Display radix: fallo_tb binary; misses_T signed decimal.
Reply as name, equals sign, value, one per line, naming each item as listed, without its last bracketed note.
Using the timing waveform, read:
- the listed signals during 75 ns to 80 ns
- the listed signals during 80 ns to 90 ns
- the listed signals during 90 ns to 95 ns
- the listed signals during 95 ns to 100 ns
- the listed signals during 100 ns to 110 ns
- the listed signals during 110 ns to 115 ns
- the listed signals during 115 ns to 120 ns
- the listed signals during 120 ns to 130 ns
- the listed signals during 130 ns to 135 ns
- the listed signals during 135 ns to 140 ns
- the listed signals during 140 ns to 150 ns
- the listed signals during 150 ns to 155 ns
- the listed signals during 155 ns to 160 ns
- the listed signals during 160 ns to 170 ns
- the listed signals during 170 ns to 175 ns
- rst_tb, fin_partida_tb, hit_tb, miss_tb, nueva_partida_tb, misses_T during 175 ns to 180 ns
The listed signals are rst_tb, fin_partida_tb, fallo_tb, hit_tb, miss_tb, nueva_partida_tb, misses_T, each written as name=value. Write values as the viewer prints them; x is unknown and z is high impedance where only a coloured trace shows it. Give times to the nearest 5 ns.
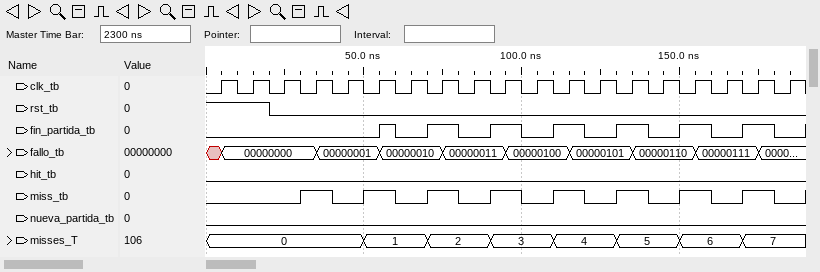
the listed signals during 75 ns to 80 ns = rst_tb=0, fin_partida_tb=1, fallo_tb=00000011, hit_tb=0, miss_tb=1, nueva_partida_tb=0, misses_T=2
the listed signals during 80 ns to 90 ns = rst_tb=0, fin_partida_tb=0, fallo_tb=00000011, hit_tb=0, miss_tb=0, nueva_partida_tb=0, misses_T=2
the listed signals during 90 ns to 95 ns = rst_tb=0, fin_partida_tb=1, fallo_tb=00000011, hit_tb=0, miss_tb=1, nueva_partida_tb=0, misses_T=3
the listed signals during 95 ns to 100 ns = rst_tb=0, fin_partida_tb=1, fallo_tb=00000100, hit_tb=0, miss_tb=1, nueva_partida_tb=0, misses_T=3
the listed signals during 100 ns to 110 ns = rst_tb=0, fin_partida_tb=0, fallo_tb=00000100, hit_tb=0, miss_tb=0, nueva_partida_tb=0, misses_T=3
the listed signals during 110 ns to 115 ns = rst_tb=0, fin_partida_tb=1, fallo_tb=00000100, hit_tb=0, miss_tb=1, nueva_partida_tb=0, misses_T=4
the listed signals during 115 ns to 120 ns = rst_tb=0, fin_partida_tb=1, fallo_tb=00000101, hit_tb=0, miss_tb=1, nueva_partida_tb=0, misses_T=4
the listed signals during 120 ns to 130 ns = rst_tb=0, fin_partida_tb=0, fallo_tb=00000101, hit_tb=0, miss_tb=0, nueva_partida_tb=0, misses_T=4
the listed signals during 130 ns to 135 ns = rst_tb=0, fin_partida_tb=1, fallo_tb=00000101, hit_tb=0, miss_tb=1, nueva_partida_tb=0, misses_T=5
the listed signals during 135 ns to 140 ns = rst_tb=0, fin_partida_tb=1, fallo_tb=00000110, hit_tb=0, miss_tb=1, nueva_partida_tb=0, misses_T=5
the listed signals during 140 ns to 150 ns = rst_tb=0, fin_partida_tb=0, fallo_tb=00000110, hit_tb=0, miss_tb=0, nueva_partida_tb=0, misses_T=5
the listed signals during 150 ns to 155 ns = rst_tb=0, fin_partida_tb=1, fallo_tb=00000110, hit_tb=0, miss_tb=1, nueva_partida_tb=0, misses_T=6
the listed signals during 155 ns to 160 ns = rst_tb=0, fin_partida_tb=1, fallo_tb=00000111, hit_tb=0, miss_tb=1, nueva_partida_tb=0, misses_T=6
the listed signals during 160 ns to 170 ns = rst_tb=0, fin_partida_tb=0, fallo_tb=00000111, hit_tb=0, miss_tb=0, nueva_partida_tb=0, misses_T=6
the listed signals during 170 ns to 175 ns = rst_tb=0, fin_partida_tb=1, fallo_tb=00000111, hit_tb=0, miss_tb=1, nueva_partida_tb=0, misses_T=7
rst_tb, fin_partida_tb, hit_tb, miss_tb, nueva_partida_tb, misses_T during 175 ns to 180 ns = rst_tb=0, fin_partida_tb=1, hit_tb=0, miss_tb=1, nueva_partida_tb=0, misses_T=7
